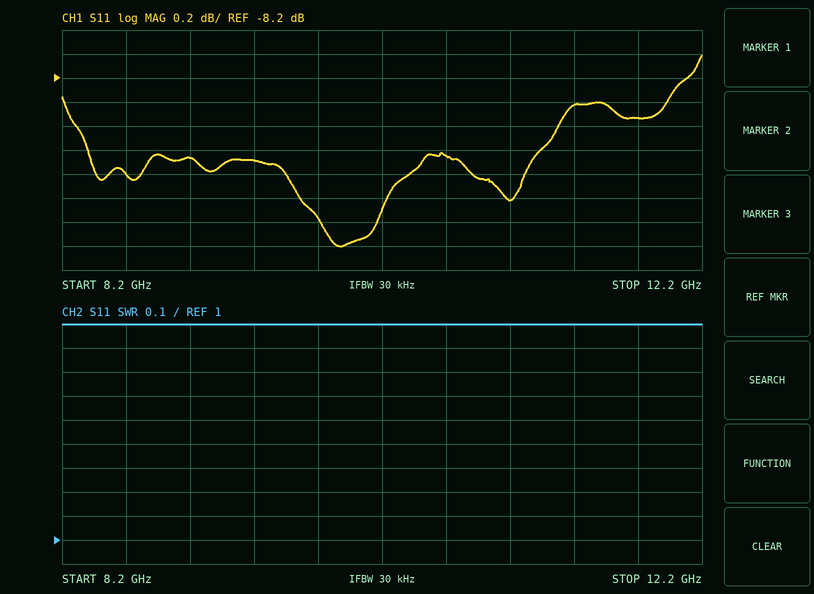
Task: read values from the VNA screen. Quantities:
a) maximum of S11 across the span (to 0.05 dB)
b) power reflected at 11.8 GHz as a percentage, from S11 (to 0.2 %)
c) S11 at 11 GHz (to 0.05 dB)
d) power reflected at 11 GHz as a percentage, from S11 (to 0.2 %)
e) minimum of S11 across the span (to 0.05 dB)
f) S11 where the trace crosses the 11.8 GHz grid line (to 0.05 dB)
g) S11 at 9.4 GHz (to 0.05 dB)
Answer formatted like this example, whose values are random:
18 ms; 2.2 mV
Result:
-8.00 dB; 14.0 %; -9.20 dB; 12.0 %; -9.60 dB; -8.55 dB; -8.90 dB
